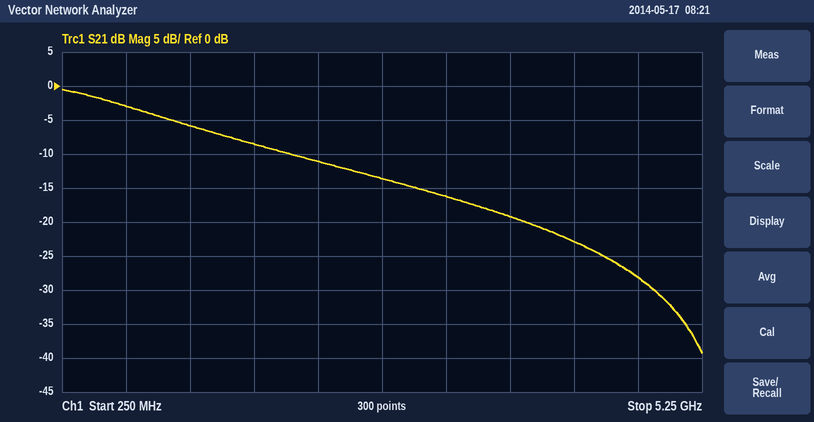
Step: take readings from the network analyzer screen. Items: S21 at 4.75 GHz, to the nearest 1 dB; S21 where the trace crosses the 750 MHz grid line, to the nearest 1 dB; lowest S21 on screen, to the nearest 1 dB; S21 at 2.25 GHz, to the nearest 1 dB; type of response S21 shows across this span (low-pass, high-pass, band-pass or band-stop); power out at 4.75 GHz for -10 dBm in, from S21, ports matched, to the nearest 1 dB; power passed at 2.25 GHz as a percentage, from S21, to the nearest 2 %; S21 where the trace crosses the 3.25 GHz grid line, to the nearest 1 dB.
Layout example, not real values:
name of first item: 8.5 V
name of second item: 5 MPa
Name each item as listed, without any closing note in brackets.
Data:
S21 at 4.75 GHz, to the nearest 1 dB: -28 dB
S21 where the trace crosses the 750 MHz grid line, to the nearest 1 dB: -3 dB
lowest S21 on screen, to the nearest 1 dB: -39 dB
S21 at 2.25 GHz, to the nearest 1 dB: -11 dB
type of response S21 shows across this span: low-pass
power out at 4.75 GHz for -10 dBm in, from S21, ports matched, to the nearest 1 dB: -38 dBm
power passed at 2.25 GHz as a percentage, from S21, to the nearest 2 %: 8 %
S21 where the trace crosses the 3.25 GHz grid line, to the nearest 1 dB: -16 dB
